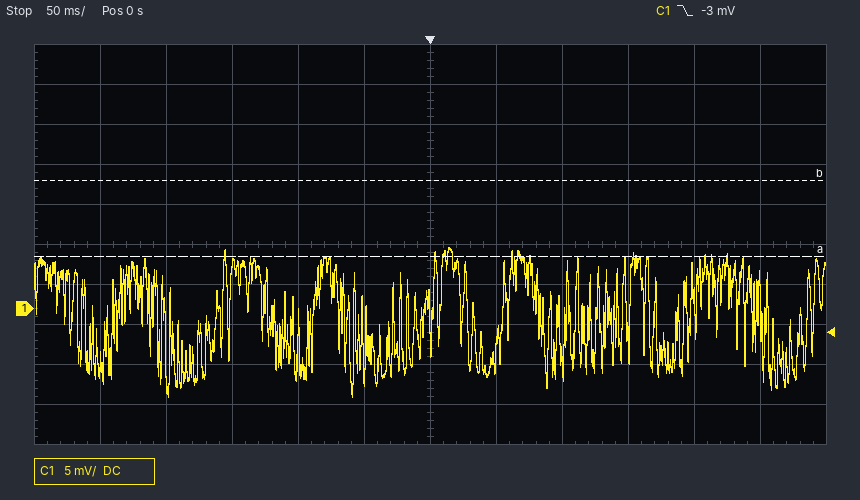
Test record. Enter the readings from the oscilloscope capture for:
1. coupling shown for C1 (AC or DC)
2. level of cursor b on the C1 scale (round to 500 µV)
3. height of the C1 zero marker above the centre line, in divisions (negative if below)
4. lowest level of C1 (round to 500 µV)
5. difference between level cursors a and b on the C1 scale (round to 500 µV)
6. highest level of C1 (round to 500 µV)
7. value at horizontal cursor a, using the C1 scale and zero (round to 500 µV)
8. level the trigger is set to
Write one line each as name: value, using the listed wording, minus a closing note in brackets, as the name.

coupling shown for C1: DC
level of cursor b on the C1 scale: 16.0 mV
height of the C1 zero marker above the centre line, in divisions: -1.6 div
lowest level of C1: -11.0 mV
difference between level cursors a and b on the C1 scale: 9.5 mV
highest level of C1: 7.5 mV
value at horizontal cursor a, using the C1 scale and zero: 6.5 mV
level the trigger is set to: -3 mV
